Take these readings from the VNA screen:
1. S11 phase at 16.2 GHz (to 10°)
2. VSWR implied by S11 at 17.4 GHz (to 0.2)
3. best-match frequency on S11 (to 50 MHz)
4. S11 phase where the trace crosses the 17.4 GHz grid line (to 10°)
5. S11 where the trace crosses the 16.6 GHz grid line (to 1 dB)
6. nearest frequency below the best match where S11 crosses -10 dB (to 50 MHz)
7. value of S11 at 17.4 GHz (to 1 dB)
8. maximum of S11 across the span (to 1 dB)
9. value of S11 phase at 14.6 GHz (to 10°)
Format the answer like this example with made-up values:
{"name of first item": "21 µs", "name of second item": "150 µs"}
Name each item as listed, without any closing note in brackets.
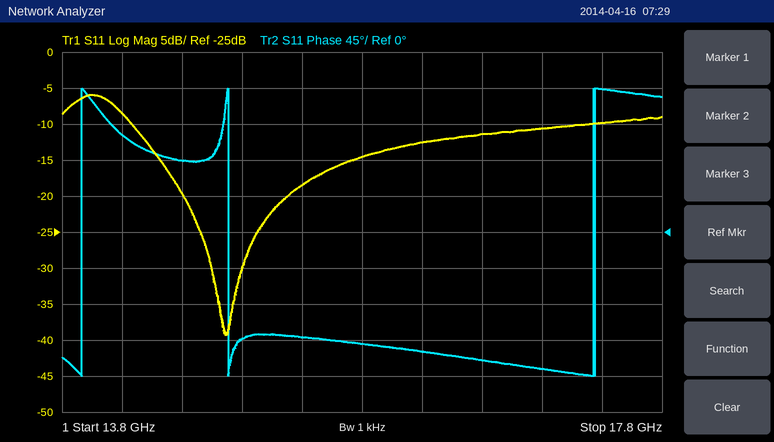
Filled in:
{"S11 phase at 16.2 GHz": "-150°", "VSWR implied by S11 at 17.4 GHz": "2.0", "best-match frequency on S11": "14.90 GHz", "S11 phase where the trace crosses the 17.4 GHz grid line": "180°", "S11 where the trace crosses the 16.6 GHz grid line": "-11 dB", "nearest frequency below the best match where S11 crosses -10 dB": "14.25 GHz", "value of S11 at 17.4 GHz": "-10 dB", "maximum of S11 across the span": "-6 dB", "value of S11 phase at 14.6 GHz": "90°"}
